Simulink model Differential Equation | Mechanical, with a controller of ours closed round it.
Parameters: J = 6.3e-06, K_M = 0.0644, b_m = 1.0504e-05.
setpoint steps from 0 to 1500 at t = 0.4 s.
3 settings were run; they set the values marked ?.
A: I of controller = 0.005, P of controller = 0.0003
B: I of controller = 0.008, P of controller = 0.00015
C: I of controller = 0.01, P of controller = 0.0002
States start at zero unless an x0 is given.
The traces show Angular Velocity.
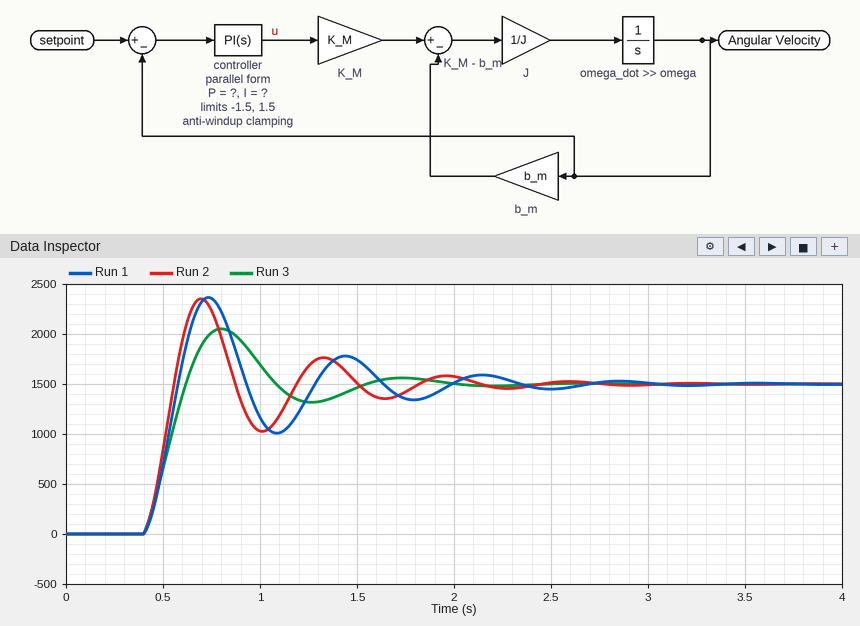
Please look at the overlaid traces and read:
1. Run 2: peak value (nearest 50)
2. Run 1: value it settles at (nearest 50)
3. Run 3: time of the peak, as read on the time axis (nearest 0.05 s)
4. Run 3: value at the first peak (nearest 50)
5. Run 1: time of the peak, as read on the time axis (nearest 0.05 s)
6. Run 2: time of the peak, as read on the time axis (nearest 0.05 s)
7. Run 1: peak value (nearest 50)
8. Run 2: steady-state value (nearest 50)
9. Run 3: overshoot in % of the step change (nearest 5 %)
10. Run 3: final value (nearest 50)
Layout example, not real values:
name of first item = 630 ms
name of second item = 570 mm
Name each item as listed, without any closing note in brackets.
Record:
Run 2: peak value = 2350
Run 1: value it settles at = 1500
Run 3: time of the peak, as read on the time axis = 0.80 s
Run 3: value at the first peak = 2050
Run 1: time of the peak, as read on the time axis = 0.75 s
Run 2: time of the peak, as read on the time axis = 0.70 s
Run 1: peak value = 2350
Run 2: steady-state value = 1500
Run 3: overshoot in % of the step change = 35 %
Run 3: final value = 1500
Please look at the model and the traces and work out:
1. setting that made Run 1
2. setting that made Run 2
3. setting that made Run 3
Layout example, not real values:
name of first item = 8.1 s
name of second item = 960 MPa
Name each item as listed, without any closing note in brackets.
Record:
setting that made Run 1 = B
setting that made Run 2 = C
setting that made Run 3 = A
